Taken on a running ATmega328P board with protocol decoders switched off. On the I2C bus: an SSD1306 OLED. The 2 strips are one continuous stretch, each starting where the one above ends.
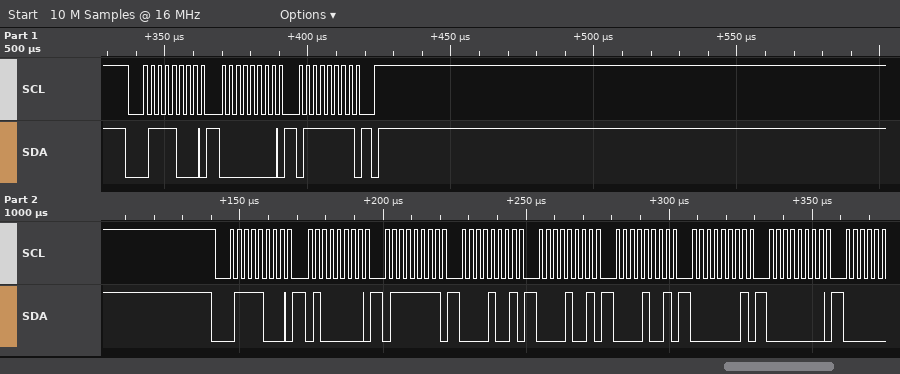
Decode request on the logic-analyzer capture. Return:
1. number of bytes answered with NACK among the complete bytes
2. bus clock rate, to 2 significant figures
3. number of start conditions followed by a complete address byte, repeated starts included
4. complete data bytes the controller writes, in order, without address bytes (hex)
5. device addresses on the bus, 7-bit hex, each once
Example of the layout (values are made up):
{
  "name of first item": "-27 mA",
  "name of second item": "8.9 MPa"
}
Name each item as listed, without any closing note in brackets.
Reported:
{
  "number of bytes answered with NACK among the complete bytes": "0",
  "bus clock rate, to 2 significant figures": "400 kHz",
  "number of start conditions followed by a complete address byte, repeated starts included": "2",
  "complete data bytes the controller writes, in order, without address bytes": "00 7F 40 7F 09 09 09 01 00",
  "device addresses on the bus, 7-bit hex, each once": "0x3C"
}
